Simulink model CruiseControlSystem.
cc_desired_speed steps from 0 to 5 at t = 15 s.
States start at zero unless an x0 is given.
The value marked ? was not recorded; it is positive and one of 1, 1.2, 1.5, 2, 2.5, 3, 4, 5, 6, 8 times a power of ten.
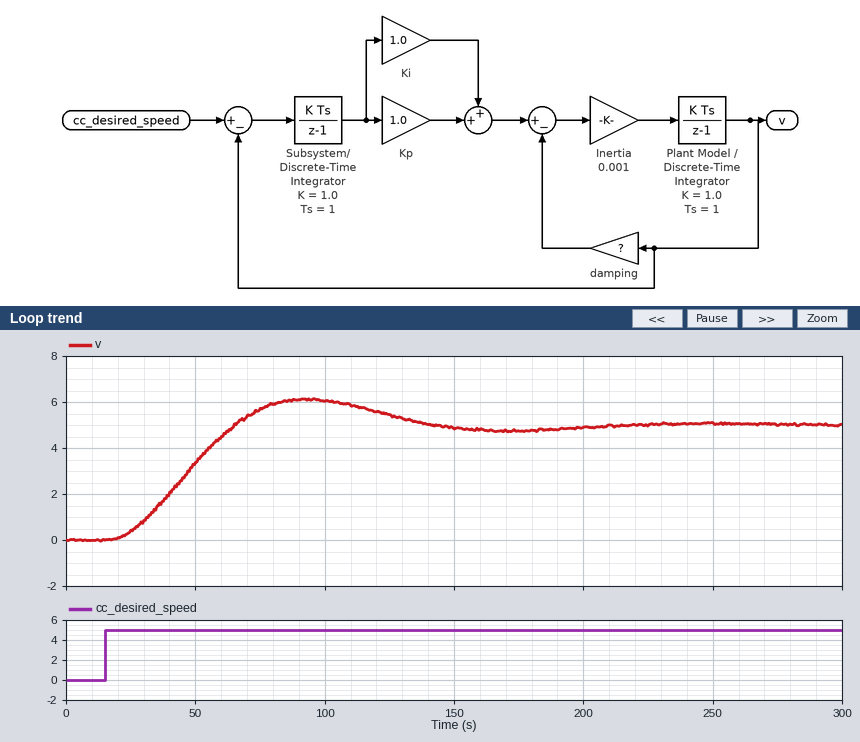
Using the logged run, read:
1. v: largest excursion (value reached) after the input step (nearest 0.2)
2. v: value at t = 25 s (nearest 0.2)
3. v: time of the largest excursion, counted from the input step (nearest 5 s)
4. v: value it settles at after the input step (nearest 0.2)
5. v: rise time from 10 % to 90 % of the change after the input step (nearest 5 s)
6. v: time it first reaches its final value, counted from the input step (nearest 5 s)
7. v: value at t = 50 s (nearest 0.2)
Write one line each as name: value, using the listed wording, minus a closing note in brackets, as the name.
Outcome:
v: largest excursion (value reached) after the input step: 6.2
v: value at t = 25 s: 0.4
v: time of the largest excursion, counted from the input step: 80 s
v: value it settles at after the input step: 5.0
v: rise time from 10 % to 90 % of the change after the input step: 35 s
v: time it first reaches its final value, counted from the input step: 50 s
v: value at t = 50 s: 3.4
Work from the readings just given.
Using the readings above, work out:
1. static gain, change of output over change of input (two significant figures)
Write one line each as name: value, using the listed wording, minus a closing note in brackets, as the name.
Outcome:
static gain, change of output over change of input: 1.0
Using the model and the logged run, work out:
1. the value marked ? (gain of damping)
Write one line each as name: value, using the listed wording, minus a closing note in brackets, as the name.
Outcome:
the value marked ?: 40
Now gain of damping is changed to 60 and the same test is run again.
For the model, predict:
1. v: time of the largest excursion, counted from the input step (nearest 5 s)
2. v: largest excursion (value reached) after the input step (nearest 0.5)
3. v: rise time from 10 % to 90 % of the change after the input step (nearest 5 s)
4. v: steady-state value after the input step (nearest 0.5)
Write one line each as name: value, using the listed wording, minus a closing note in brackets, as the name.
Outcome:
v: time of the largest excursion, counted from the input step: 90 s
v: largest excursion (value reached) after the input step: 5.5
v: rise time from 10 % to 90 % of the change after the input step: 45 s
v: steady-state value after the input step: 5.0
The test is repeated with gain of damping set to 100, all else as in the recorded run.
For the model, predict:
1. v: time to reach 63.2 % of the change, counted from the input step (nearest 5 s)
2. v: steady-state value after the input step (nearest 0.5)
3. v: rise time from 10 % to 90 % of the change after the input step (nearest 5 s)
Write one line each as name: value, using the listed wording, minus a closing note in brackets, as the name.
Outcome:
v: time to reach 63.2 % of the change, counted from the input step: 50 s
v: steady-state value after the input step: 5.0
v: rise time from 10 % to 90 % of the change after the input step: 85 s
